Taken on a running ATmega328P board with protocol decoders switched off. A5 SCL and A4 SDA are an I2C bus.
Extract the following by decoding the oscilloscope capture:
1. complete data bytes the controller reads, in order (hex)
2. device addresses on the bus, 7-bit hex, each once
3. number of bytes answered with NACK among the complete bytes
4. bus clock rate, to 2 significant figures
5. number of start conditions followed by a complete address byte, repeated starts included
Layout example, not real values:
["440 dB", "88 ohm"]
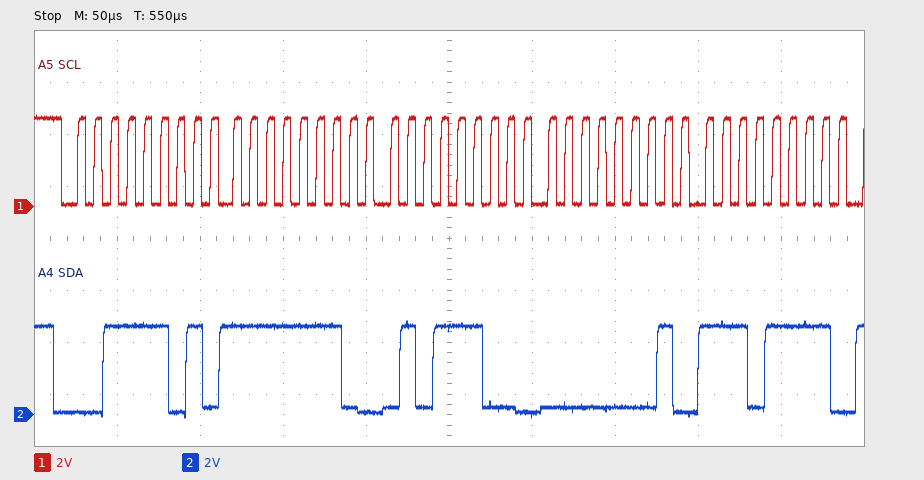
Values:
["FE 5C 01 EF", "0x1E", "0", "100 kHz", "1"]
